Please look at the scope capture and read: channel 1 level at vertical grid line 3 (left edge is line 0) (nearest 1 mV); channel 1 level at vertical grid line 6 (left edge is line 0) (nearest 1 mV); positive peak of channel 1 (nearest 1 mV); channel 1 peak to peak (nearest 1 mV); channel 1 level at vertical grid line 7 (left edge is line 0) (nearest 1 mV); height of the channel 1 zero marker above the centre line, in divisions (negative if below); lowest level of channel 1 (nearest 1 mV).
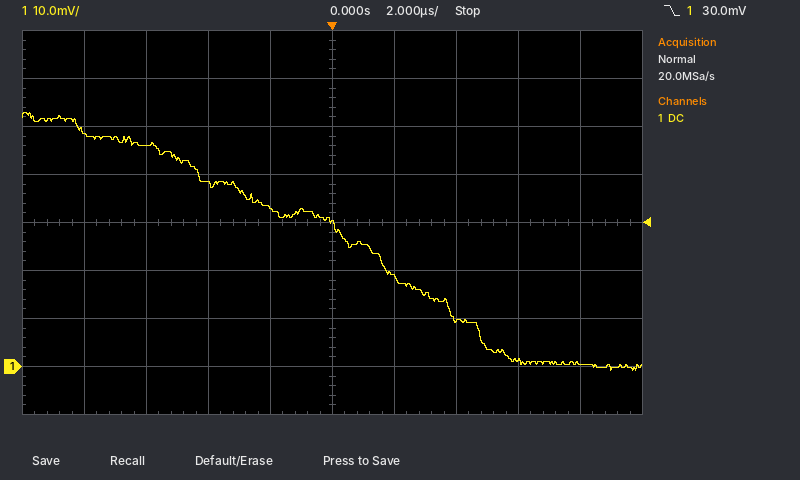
38 mV
19 mV
53 mV
54 mV
10 mV
-3.0 div
-1 mV
